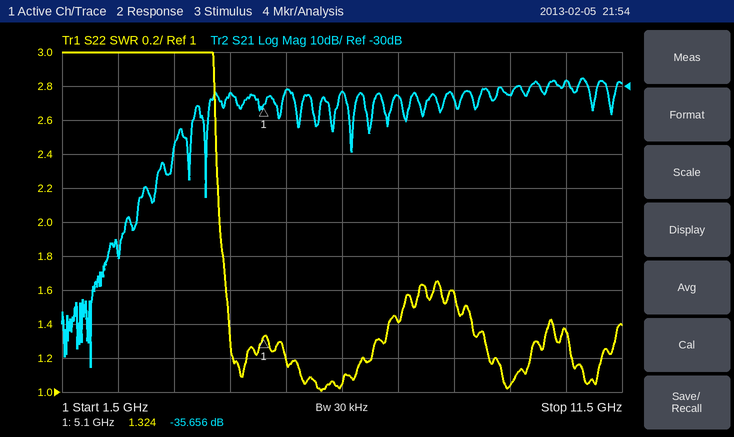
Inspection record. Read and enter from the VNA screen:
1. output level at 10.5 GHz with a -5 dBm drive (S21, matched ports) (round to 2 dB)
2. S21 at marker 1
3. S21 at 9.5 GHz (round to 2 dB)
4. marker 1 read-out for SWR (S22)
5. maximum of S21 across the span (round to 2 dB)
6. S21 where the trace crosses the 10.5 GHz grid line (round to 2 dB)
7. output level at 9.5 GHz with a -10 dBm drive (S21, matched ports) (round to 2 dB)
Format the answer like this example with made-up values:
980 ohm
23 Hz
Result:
-34 dBm
-35.656 dB
-32 dB
1.324
-28 dB
-28 dB
-42 dBm
